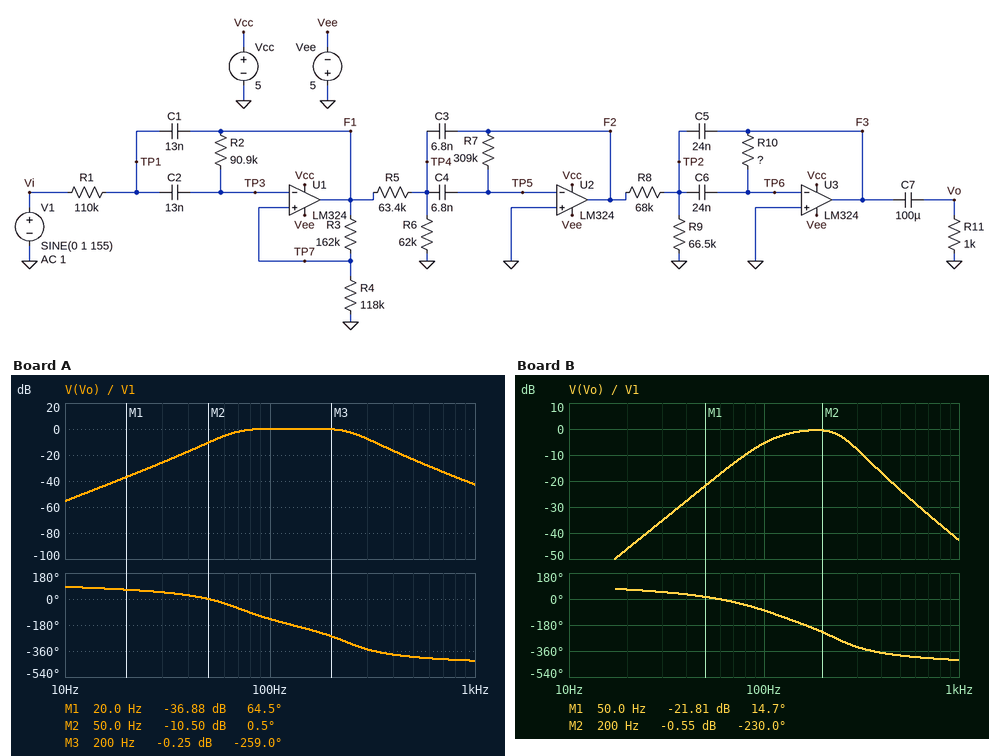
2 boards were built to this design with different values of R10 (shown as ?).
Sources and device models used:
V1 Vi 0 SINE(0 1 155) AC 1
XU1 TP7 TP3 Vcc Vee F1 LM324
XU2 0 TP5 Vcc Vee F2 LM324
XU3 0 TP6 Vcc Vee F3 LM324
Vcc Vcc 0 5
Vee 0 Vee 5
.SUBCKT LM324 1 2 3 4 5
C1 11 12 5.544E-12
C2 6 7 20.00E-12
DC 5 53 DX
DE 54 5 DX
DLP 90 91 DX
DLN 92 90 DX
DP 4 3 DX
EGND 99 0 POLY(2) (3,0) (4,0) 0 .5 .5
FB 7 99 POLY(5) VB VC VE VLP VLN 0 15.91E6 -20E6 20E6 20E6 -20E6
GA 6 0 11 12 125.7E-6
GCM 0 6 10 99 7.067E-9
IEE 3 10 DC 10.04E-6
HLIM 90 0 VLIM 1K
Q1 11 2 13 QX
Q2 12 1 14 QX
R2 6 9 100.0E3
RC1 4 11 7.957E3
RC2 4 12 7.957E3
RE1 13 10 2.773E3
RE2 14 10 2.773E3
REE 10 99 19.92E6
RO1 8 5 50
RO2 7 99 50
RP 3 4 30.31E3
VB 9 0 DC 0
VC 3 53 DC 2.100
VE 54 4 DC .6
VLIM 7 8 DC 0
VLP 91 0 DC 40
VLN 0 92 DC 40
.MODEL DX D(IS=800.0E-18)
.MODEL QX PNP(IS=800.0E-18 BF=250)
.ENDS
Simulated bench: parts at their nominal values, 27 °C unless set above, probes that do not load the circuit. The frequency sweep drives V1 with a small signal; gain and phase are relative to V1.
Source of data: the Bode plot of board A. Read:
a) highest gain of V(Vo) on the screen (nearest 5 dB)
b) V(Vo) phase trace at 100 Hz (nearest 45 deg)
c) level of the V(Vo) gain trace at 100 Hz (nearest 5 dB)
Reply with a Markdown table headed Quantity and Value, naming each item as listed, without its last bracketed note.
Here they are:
| Quantity | Value |
|---|---|
| highest gain of V(Vo) on the screen | 0 dB |
| V(Vo) phase trace at 100 Hz | -135 deg |
| level of the V(Vo) gain trace at 100 Hz | 0 dB |
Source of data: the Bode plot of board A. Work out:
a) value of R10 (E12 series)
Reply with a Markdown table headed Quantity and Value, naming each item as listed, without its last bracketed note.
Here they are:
| Quantity | Value |
|---|---|
| value of R10 | 270 kΩ |
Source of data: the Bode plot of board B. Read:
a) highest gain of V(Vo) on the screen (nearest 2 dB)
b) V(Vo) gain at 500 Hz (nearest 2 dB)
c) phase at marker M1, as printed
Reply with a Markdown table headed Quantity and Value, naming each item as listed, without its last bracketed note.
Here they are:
| Quantity | Value |
|---|---|
| highest gain of V(Vo) on the screen | 0 dB |
| V(Vo) gain at 500 Hz | -24 dB |
| phase at marker M1, as printed | 14.7 deg |
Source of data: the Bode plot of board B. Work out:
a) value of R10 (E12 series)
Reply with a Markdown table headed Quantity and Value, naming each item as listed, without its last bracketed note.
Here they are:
| Quantity | Value |
|---|---|
| value of R10 | 100 kΩ |
